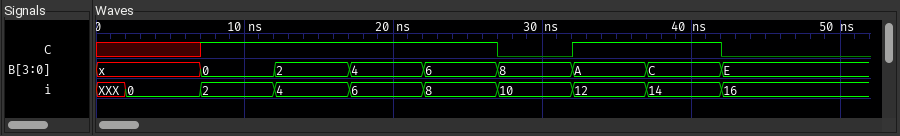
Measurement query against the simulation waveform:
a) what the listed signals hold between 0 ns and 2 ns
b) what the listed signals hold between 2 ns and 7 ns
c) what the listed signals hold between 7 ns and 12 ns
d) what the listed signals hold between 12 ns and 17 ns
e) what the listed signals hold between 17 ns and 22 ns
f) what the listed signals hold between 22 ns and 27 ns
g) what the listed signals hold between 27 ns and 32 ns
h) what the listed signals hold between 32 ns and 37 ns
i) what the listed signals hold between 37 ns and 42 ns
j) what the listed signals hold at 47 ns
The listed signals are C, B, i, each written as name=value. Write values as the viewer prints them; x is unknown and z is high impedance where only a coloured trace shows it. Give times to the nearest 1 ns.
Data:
C=x, B=x, i=XXX
C=x, B=x, i=0
C=1, B=0, i=2
C=1, B=2, i=4
C=1, B=4, i=6
C=1, B=6, i=8
C=0, B=8, i=10
C=1, B=A, i=12
C=1, B=C, i=14
C=0, B=E, i=16
